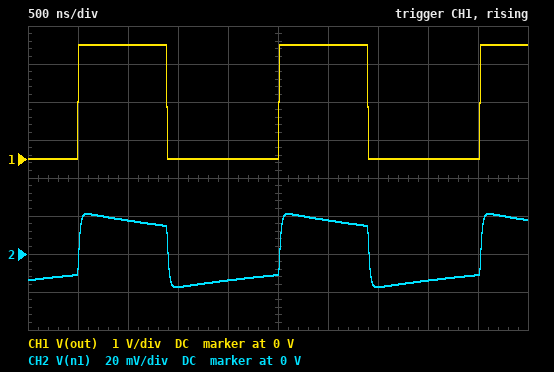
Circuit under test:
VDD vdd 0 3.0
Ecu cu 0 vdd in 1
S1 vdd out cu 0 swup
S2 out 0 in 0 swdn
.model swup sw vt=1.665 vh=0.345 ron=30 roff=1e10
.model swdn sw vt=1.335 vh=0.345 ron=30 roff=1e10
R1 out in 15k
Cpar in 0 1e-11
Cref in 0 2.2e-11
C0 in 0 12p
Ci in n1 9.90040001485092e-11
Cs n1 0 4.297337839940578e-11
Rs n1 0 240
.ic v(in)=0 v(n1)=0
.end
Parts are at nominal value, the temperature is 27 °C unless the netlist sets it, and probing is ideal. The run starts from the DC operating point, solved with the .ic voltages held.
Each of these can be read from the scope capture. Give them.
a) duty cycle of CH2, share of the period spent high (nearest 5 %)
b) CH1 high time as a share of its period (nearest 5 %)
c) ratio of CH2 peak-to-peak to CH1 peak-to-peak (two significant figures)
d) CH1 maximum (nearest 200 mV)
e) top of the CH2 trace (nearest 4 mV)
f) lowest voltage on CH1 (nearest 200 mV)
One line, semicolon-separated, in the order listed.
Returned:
45 %; 45 %; 0.013; 3.0 V; 20 mV; 0 V
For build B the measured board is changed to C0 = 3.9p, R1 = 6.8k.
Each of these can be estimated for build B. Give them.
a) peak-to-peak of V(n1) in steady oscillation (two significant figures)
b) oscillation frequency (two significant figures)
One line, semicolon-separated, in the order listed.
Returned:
85 mV; 1.2 MHz
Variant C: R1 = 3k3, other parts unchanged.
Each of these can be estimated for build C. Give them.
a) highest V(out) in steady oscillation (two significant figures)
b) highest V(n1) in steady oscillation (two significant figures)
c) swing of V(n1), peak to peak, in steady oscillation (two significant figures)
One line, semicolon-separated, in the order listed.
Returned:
3.0 V; 83 mV; 150 mV
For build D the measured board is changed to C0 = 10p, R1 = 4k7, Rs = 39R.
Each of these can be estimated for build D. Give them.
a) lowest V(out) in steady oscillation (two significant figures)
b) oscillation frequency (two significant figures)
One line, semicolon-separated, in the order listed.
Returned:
6.3 mV; 1.6 MHz
